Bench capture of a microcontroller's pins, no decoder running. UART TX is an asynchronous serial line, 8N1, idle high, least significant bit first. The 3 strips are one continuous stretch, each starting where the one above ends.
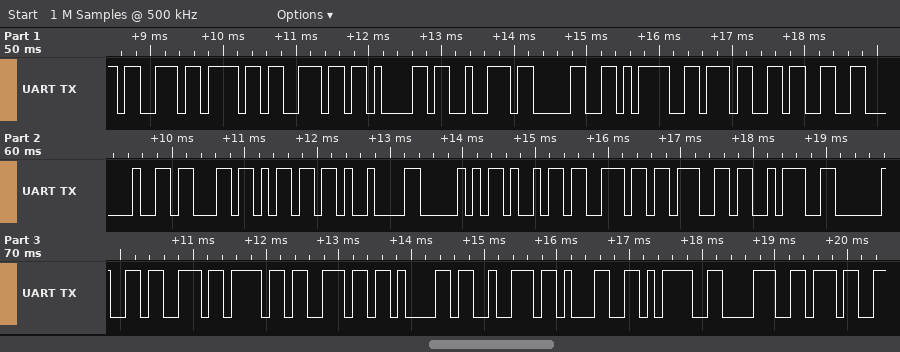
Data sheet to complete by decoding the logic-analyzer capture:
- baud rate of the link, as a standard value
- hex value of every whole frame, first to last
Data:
9600 baud
73 6F 6E 61 72 30 3D 37 33 20 63 6D 09 50 69 6E 67 3A 20 73 6F 6E 61 72 31 3D 38 37
